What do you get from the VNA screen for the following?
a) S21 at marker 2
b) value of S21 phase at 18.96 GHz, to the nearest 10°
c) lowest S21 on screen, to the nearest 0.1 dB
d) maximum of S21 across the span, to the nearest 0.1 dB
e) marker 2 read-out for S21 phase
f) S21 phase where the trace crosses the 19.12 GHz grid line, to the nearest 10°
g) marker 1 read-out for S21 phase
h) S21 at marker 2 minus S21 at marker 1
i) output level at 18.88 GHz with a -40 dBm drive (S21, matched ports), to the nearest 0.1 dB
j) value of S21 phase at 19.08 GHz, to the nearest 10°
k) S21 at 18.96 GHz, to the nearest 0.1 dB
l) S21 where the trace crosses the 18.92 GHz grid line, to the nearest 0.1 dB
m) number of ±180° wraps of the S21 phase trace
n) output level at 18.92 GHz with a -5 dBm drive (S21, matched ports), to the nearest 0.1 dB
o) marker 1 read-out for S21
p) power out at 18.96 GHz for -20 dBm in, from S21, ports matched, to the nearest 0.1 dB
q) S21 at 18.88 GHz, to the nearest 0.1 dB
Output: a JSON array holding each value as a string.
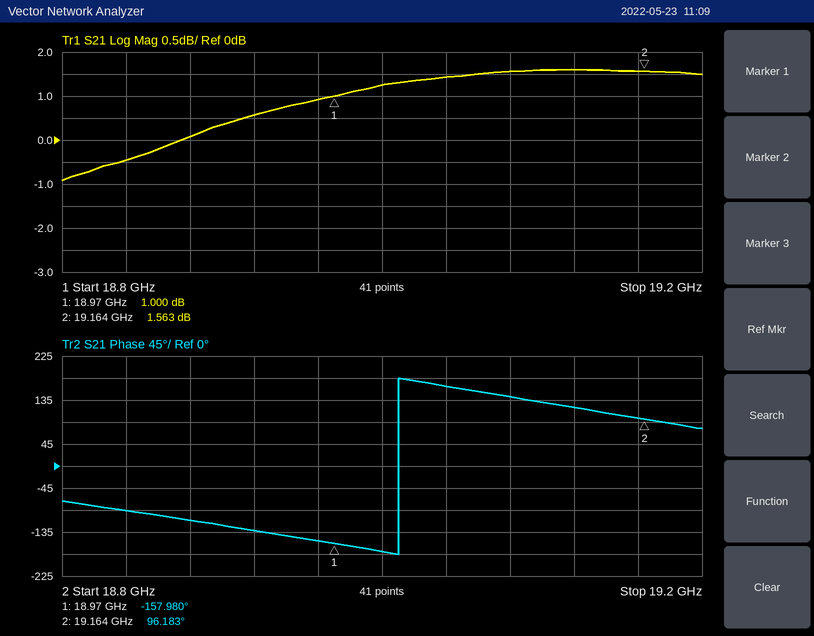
["1.563 dB", "-150°", "-0.9 dB", "1.6 dB", "96.183°", "120°", "-157.980°", "0.563 dB", "-39.9 dBm", "140°", "0.9 dB", "0.6 dB", "1", "-4.4 dBm", "1.000 dB", "-19.1 dBm", "0.1 dB"]
